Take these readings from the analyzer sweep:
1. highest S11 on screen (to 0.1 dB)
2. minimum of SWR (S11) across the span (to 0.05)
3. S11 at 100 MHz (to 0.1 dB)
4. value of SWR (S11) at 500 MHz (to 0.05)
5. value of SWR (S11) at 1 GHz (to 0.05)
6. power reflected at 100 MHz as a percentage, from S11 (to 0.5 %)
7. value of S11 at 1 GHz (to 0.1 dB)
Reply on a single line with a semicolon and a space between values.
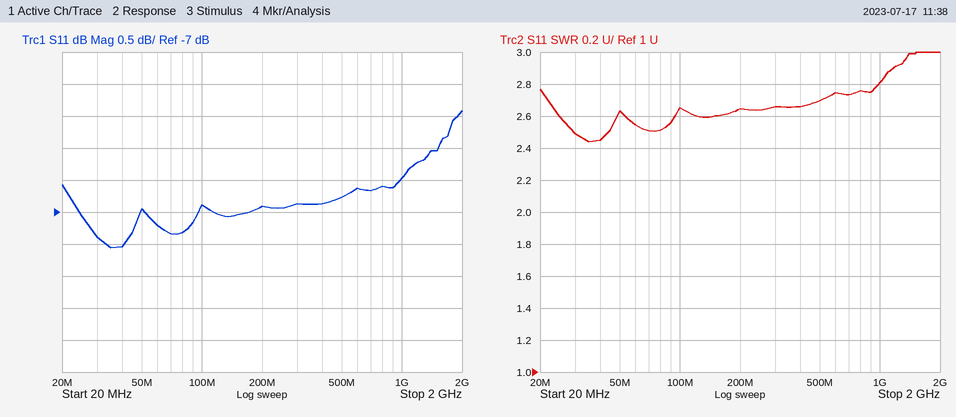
-5.4 dB; 2.45; -6.9 dB; 2.70; 2.80; 20.5 %; -6.5 dB
